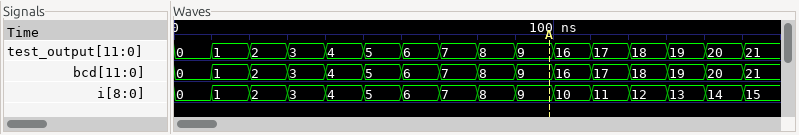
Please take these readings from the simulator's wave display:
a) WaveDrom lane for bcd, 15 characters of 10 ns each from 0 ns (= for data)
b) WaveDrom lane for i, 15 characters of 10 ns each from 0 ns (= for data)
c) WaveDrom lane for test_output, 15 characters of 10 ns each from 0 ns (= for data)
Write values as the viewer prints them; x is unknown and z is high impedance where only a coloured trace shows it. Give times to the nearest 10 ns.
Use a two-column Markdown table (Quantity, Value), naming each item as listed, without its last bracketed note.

| Quantity | Value |
|---|---|
| WaveDrom lane for bcd, 15 characters of 10 ns each from 0 ns | {name: 'bcd', wave: '===============', data: '0 1 2 3 4 5 6 7 8 9 16 17 18 19 20'} |
| WaveDrom lane for i, 15 characters of 10 ns each from 0 ns | {name: 'i', wave: '===============', data: '0 1 2 3 4 5 6 7 8 9 10 11 12 13 14'} |
| WaveDrom lane for test_output, 15 characters of 10 ns each from 0 ns | {name: 'test_output', wave: '===============', data: '0 1 2 3 4 5 6 7 8 9 16 17 18 19 20'} |
